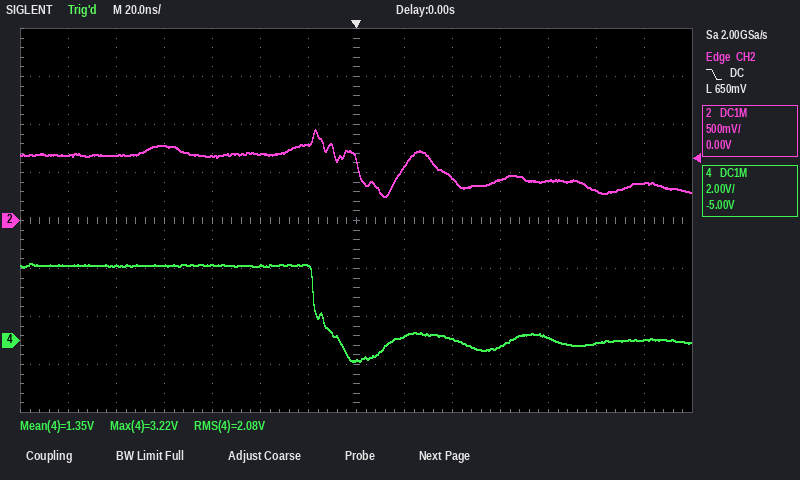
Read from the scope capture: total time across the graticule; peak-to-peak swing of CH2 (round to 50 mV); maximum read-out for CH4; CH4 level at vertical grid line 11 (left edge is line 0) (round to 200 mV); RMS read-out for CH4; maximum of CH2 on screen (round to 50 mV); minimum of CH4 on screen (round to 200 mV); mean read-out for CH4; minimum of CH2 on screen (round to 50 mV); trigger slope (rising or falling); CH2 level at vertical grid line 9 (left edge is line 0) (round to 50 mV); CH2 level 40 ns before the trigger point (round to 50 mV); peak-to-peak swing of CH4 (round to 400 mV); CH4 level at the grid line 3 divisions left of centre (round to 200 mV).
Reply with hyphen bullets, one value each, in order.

- 280 ns
- 700 mV
- 3.22 V
- 200 mV
- 2.08 V
- 950 mV
- -800 mV
- 1.35 V
- 250 mV
- falling
- 450 mV
- 700 mV
- 4.0 V
- 3.2 V
